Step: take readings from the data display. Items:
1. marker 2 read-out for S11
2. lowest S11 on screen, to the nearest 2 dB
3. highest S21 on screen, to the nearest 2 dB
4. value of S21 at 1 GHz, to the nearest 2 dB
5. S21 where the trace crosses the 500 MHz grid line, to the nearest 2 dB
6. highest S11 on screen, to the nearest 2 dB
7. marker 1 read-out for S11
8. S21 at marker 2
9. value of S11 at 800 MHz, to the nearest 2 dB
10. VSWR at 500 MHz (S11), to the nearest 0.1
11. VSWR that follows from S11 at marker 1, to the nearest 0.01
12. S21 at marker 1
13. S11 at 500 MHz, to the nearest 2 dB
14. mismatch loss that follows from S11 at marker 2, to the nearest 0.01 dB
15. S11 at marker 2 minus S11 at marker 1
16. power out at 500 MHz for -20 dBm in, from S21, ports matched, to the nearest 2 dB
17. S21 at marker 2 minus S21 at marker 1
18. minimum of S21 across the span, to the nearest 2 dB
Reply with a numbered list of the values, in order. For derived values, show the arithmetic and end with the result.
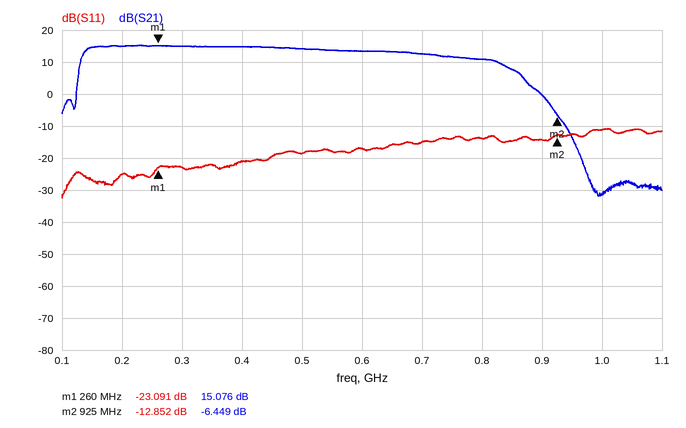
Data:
1. -12.852 dB
2. -32 dB
3. 16 dB
4. -32 dB
5. 14 dB
6. -10 dB
7. -23.091 dB
8. -6.449 dB
9. -14 dB
10. |Γ| = 10^(-18/20) = 0.1259; VSWR = (1 + 0.1259)/(1 − 0.1259) ≈ 1.3
11. (1 + 0.0701)/(1 − 0.0701) ≈ 1.15
12. 15.076 dB
13. -18 dB
14. −10 log10(1 − 10^(-12.852/10)) ≈ 0.23 dB
15. -12.852 − (-23.091) = 10.239 dB
16. -20 dBm + (14 dB) = -6 dBm
17. -6.449 − (15.076) = -21.525 dB
18. -32 dB
